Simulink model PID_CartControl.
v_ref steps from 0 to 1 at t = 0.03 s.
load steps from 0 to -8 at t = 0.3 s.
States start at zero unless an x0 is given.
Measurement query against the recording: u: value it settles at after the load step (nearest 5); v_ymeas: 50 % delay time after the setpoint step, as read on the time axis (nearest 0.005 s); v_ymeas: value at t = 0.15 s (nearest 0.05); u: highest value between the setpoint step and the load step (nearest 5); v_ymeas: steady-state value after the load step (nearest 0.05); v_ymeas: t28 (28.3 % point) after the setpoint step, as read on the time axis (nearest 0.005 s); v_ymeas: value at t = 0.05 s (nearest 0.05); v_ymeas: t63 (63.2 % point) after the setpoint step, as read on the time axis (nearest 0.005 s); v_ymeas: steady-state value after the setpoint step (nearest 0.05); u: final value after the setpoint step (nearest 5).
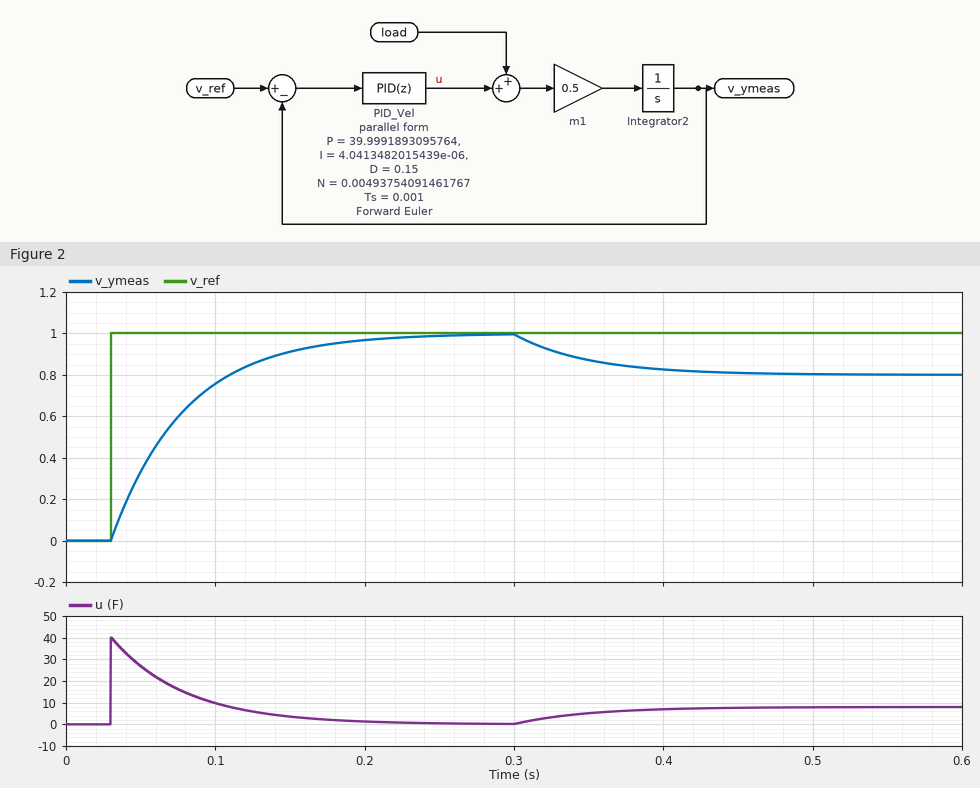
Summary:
10
0.065 s
0.90
40
0.80
0.045 s
0.35
0.080 s
1.00
0
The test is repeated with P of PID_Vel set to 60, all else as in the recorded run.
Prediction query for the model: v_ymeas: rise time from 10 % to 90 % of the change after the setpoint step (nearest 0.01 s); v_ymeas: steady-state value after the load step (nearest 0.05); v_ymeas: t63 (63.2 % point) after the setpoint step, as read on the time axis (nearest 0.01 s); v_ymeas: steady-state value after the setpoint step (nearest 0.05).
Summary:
0.07 s
0.85
0.06 s
1.00
